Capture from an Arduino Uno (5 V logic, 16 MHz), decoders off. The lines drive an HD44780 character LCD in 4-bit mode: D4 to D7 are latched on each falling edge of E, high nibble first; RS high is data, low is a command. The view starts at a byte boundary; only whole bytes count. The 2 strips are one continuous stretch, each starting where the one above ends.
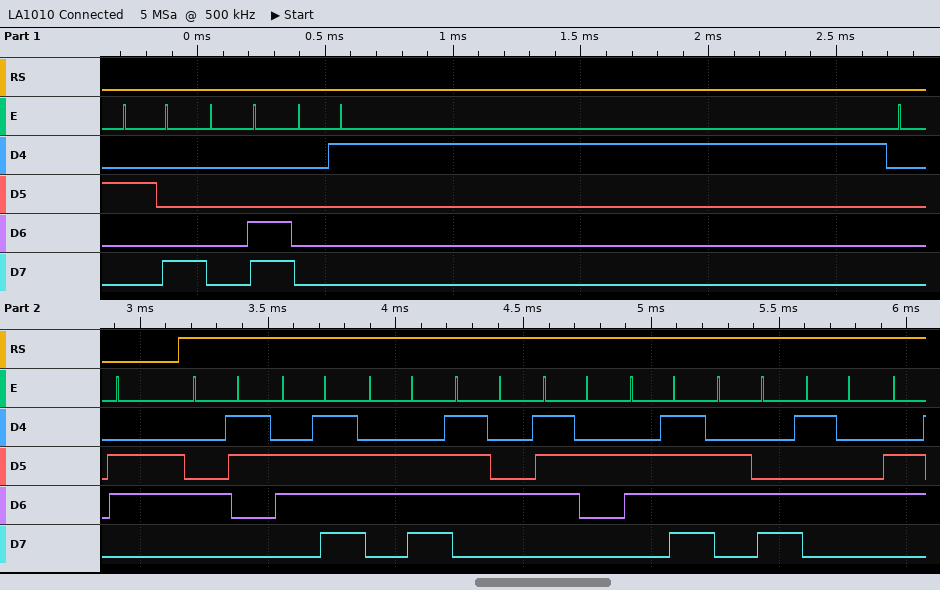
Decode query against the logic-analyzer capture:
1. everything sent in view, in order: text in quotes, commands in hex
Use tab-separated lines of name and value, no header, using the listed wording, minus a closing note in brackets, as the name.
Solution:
everything sent in view, in order: text in quotes, commands in hex	0x28 0x0C 0x01 0x06 "ControlT"
